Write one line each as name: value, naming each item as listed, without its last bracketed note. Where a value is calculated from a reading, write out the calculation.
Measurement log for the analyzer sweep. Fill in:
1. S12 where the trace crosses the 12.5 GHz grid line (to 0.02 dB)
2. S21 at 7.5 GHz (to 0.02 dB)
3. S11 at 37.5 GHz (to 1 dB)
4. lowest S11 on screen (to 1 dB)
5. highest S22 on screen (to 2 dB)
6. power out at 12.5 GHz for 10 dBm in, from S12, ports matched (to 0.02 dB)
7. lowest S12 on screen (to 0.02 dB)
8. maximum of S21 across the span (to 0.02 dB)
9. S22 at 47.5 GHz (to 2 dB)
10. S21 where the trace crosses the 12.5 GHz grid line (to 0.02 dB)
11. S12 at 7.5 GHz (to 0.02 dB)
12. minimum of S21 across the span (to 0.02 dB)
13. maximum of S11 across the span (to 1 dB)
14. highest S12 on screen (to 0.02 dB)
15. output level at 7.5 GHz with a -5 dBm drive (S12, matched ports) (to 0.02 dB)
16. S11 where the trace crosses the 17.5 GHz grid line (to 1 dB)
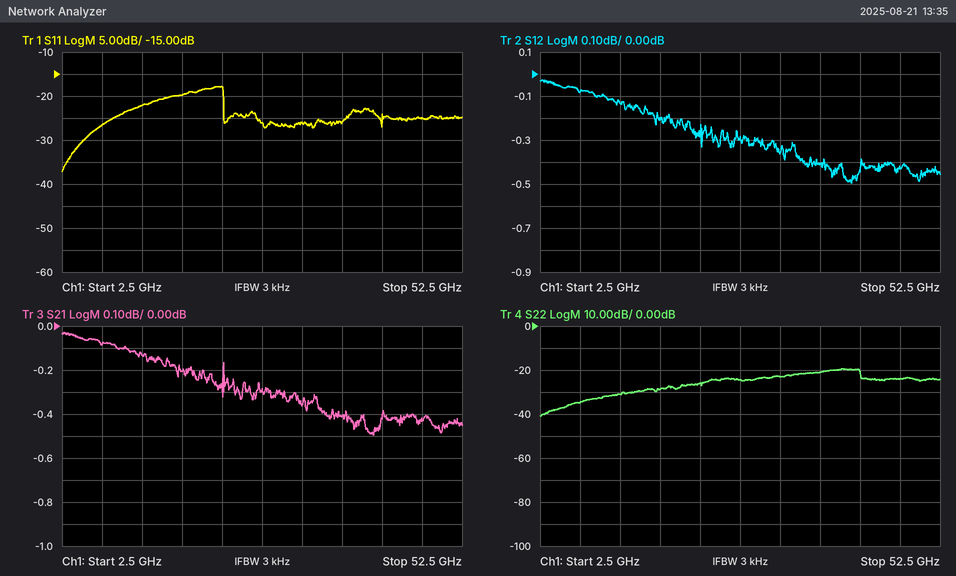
S12 where the trace crosses the 12.5 GHz grid line: -0.14 dB
S21 at 7.5 GHz: -0.08 dB
S11 at 37.5 GHz: -26 dB
lowest S11 on screen: -37 dB
highest S22 on screen: -20 dB
power out at 12.5 GHz for 10 dBm in, from S12, ports matched: 10 dBm + (-0.14 dB) = 9.86 dBm
lowest S12 on screen: -0.50 dB
maximum of S21 across the span: -0.02 dB
S22 at 47.5 GHz: -24 dB
S21 where the trace crosses the 12.5 GHz grid line: -0.14 dB
S12 at 7.5 GHz: -0.08 dB
minimum of S21 across the span: -0.50 dB
maximum of S11 across the span: -18 dB
highest S12 on screen: -0.02 dB
output level at 7.5 GHz with a -5 dBm drive (S12, matched ports): -5 dBm + (-0.08 dB) = -5.08 dBm
S11 where the trace crosses the 17.5 GHz grid line: -20 dB
